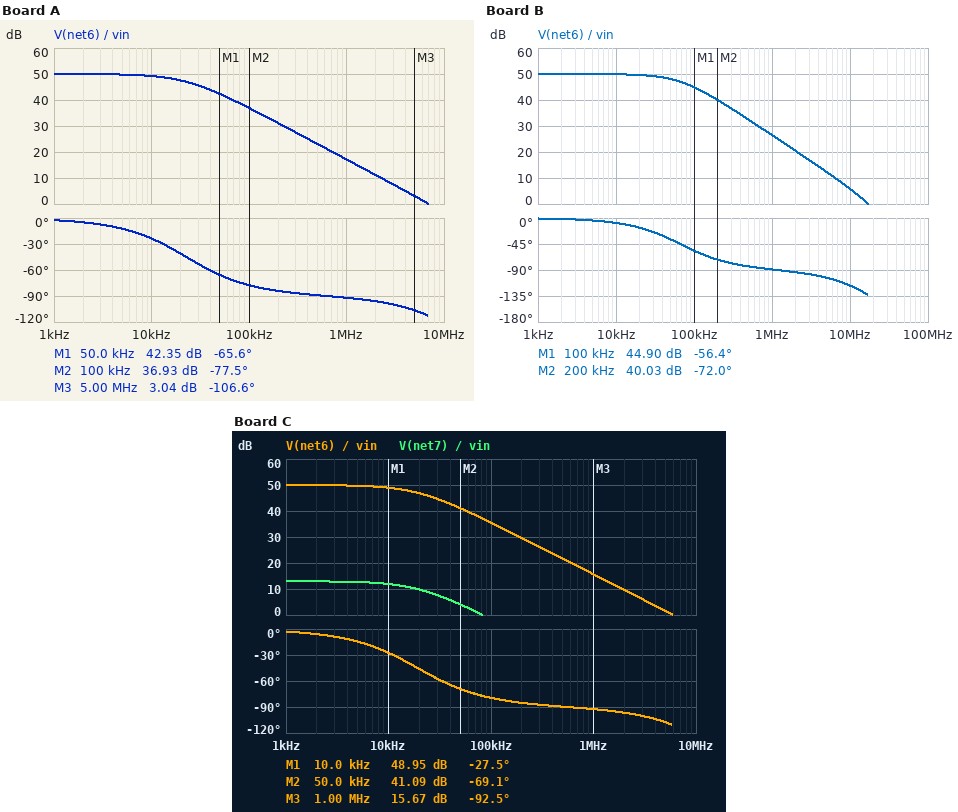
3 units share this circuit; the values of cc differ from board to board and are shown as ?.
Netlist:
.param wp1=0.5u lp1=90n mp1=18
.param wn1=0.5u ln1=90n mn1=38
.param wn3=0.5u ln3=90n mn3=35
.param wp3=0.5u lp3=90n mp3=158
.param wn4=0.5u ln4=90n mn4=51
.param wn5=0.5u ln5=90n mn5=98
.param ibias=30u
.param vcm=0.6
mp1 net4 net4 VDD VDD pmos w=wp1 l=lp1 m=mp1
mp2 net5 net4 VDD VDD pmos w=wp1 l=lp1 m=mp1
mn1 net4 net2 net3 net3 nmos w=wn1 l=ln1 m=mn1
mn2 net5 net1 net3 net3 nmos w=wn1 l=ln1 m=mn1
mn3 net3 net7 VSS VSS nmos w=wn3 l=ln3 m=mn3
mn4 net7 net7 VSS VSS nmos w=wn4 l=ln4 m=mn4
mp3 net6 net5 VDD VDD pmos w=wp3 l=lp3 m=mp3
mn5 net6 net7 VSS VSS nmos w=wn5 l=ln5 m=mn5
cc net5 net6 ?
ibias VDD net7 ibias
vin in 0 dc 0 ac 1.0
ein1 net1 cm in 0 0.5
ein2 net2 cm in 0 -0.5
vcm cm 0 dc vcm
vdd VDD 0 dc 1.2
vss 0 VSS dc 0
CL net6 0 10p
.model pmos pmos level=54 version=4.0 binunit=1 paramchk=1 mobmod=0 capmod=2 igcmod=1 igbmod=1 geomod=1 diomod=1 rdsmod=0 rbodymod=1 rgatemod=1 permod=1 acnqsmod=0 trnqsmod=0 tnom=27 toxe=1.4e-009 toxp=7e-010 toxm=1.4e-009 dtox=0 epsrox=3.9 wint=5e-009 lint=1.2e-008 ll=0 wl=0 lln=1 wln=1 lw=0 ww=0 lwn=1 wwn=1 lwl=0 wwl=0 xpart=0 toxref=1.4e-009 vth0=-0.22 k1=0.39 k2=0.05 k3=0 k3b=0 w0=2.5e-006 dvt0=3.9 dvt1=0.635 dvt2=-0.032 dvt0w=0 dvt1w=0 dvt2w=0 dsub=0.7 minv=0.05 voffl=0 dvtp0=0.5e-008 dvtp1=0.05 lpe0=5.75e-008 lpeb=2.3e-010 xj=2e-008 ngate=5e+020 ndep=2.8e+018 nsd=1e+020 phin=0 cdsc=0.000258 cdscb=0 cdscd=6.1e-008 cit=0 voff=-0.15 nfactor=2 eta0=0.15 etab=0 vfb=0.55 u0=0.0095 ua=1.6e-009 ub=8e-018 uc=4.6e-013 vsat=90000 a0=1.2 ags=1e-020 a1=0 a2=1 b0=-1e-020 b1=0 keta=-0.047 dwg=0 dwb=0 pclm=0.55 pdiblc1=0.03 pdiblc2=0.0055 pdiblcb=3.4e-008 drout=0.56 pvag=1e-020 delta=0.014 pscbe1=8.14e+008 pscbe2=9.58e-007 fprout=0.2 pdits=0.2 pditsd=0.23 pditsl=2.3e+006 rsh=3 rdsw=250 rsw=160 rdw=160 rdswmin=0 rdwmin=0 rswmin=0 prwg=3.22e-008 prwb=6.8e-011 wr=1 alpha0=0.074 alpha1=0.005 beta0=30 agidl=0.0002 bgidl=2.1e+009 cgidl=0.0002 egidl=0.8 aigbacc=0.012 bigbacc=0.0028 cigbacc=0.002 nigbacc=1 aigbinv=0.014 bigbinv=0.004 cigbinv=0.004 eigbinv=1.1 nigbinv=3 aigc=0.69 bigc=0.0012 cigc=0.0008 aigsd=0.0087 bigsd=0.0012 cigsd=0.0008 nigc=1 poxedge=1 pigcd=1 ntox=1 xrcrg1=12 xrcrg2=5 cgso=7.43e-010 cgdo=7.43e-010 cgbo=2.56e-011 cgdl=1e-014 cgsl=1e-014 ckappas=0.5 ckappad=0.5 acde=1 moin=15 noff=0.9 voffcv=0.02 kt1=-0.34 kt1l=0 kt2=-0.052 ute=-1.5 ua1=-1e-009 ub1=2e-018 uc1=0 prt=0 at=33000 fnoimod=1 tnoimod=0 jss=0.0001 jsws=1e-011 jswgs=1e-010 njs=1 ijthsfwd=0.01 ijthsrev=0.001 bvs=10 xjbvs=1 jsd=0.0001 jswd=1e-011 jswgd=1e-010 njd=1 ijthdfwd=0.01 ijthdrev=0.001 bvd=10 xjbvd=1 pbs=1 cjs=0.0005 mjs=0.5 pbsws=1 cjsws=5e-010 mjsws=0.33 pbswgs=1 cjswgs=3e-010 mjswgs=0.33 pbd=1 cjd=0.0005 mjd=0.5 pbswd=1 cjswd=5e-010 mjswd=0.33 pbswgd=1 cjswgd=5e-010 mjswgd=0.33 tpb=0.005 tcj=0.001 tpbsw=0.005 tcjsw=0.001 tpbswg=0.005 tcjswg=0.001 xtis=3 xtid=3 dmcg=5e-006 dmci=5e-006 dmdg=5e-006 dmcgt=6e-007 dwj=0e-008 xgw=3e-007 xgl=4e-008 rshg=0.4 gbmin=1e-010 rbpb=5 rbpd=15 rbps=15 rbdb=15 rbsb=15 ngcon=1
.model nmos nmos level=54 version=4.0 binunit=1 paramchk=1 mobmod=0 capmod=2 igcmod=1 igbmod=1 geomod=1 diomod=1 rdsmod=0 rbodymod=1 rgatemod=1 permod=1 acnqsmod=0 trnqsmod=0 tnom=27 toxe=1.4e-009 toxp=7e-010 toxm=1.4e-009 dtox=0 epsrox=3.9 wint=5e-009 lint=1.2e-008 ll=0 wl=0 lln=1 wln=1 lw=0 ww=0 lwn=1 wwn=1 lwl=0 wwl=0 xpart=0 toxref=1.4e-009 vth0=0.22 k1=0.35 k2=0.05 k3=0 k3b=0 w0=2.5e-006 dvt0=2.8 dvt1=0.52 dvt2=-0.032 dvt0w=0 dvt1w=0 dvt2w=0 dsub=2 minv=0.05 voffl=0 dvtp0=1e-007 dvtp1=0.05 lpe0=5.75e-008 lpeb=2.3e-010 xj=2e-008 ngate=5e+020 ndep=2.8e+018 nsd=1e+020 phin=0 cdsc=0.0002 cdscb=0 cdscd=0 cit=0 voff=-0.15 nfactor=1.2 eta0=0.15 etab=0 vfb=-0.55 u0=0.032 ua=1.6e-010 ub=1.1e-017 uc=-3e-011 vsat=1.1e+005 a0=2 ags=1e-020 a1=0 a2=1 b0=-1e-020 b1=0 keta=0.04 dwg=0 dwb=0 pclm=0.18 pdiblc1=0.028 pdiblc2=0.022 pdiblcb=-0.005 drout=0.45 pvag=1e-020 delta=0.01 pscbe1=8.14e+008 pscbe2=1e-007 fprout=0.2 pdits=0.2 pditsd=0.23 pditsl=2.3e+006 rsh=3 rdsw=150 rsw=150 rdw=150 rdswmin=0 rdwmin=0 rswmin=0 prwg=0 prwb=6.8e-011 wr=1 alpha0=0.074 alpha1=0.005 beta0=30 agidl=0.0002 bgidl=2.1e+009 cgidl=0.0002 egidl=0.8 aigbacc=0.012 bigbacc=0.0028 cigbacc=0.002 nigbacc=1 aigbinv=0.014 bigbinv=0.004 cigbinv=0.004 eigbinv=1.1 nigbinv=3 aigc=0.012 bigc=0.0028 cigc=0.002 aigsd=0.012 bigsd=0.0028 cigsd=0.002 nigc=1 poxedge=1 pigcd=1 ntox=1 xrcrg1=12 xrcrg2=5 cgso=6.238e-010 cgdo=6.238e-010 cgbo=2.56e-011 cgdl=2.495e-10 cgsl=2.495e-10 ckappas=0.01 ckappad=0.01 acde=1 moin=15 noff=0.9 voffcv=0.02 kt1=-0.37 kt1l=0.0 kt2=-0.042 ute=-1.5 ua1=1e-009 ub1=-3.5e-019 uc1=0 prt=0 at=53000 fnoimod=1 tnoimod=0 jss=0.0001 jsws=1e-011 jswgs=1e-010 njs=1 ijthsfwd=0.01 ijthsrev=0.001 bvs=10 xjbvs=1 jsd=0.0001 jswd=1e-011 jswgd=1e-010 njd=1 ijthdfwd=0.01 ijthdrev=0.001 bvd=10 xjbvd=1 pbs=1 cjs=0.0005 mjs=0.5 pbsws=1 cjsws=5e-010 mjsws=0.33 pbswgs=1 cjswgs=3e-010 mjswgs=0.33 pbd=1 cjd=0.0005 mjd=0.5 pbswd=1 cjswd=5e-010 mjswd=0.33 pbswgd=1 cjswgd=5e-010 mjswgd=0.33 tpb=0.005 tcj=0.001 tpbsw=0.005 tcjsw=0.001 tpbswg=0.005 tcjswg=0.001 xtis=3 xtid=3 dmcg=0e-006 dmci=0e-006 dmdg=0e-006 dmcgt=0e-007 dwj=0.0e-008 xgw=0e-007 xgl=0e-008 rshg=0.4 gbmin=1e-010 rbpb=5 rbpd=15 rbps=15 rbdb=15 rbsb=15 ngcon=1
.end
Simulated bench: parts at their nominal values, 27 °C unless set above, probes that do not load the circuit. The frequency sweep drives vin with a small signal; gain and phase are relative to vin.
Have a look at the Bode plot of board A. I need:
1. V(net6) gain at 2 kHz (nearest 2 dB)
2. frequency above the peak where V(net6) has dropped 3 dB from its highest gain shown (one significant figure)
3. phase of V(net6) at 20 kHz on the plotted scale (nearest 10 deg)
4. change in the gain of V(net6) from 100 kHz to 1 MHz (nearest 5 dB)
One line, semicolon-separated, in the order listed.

50 dB; 20 kHz; -40 deg; -20 dB
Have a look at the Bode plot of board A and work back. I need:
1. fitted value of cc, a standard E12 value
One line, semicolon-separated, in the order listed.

4.7 pF
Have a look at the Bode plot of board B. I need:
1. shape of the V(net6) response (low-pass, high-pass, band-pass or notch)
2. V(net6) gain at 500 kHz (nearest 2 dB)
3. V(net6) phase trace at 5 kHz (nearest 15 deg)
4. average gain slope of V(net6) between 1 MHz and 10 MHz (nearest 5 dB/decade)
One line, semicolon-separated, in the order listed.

low-pass; 32 dB; 0 deg; -20 dB/decade
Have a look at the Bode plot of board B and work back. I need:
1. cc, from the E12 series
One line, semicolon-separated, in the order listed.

1.5 pF
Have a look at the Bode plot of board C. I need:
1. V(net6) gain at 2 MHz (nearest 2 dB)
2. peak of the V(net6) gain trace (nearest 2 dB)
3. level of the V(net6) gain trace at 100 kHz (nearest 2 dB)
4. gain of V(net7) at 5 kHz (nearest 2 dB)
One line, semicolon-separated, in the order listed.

10 dB; 50 dB; 36 dB; 12 dB
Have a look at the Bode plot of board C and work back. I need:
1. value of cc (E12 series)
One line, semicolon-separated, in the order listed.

5.6 pF
